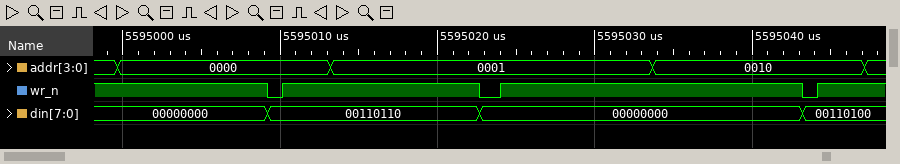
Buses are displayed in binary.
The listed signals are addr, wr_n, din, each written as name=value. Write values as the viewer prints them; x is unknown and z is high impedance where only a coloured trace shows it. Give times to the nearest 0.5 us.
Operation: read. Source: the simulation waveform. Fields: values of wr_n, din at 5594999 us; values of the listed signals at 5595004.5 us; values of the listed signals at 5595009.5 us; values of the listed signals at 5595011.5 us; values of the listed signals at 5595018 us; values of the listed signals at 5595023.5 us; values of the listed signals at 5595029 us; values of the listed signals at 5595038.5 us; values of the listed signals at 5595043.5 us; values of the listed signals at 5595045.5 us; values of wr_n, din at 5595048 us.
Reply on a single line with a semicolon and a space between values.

wr_n=1, din=00000000; addr=0000, wr_n=1, din=00000000; addr=0000, wr_n=0, din=00110110; addr=0000, wr_n=1, din=00110110; addr=0001, wr_n=1, din=00110110; addr=0001, wr_n=0, din=00000000; addr=0001, wr_n=1, din=00000000; addr=0010, wr_n=1, din=00000000; addr=0010, wr_n=0, din=00110100; addr=0010, wr_n=1, din=00110100; wr_n=1, din=00110100
